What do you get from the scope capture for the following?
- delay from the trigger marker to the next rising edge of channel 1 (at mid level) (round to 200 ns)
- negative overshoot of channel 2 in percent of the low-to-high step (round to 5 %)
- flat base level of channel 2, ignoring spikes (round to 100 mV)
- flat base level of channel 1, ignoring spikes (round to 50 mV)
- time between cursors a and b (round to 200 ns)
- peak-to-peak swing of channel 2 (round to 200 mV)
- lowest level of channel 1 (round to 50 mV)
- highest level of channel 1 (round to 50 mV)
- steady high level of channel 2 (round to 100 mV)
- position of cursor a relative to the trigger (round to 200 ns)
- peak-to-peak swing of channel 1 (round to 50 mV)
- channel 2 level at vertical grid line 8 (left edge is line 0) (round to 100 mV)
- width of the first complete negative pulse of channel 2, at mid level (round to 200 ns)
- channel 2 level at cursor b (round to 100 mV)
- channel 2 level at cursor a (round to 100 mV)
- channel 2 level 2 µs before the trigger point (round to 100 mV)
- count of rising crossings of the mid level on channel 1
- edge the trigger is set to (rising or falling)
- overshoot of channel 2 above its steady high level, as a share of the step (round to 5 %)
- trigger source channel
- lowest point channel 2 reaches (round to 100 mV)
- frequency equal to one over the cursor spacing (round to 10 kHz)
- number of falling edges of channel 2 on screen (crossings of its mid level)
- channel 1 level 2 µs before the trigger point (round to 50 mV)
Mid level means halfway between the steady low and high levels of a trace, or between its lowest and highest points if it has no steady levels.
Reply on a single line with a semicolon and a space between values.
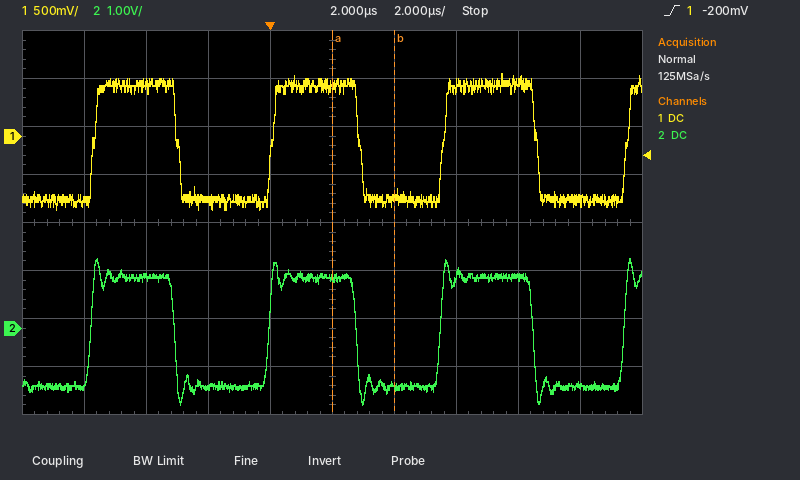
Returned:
5.6 µs; 15 %; -1.2 V; -650 mV; 2.0 µs; 3.0 V; -750 mV; 650 mV; 1.1 V; +2.0 µs; 1.40 V; 1.1 V; 3.0 µs; -1.2 V; 1.0 V; -1.2 V; 4; rising; 15 %; channel 1; -1.6 V; 500 kHz; 3; -650 mV
